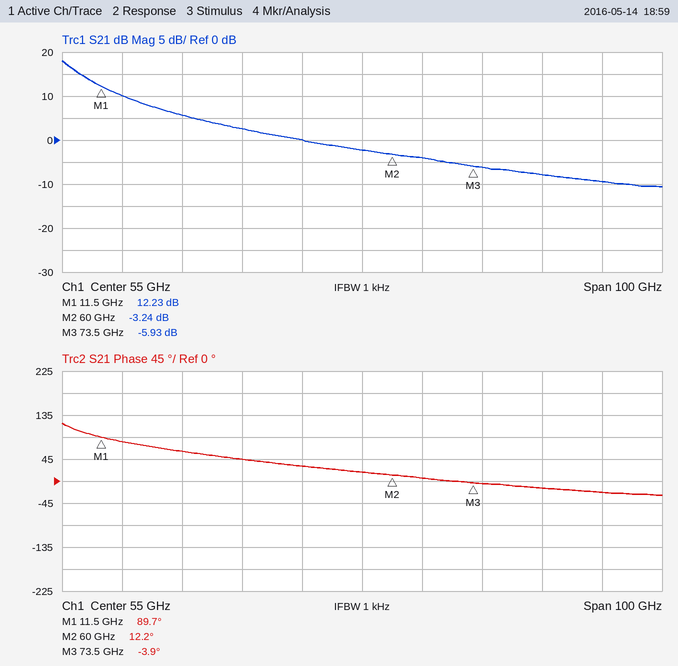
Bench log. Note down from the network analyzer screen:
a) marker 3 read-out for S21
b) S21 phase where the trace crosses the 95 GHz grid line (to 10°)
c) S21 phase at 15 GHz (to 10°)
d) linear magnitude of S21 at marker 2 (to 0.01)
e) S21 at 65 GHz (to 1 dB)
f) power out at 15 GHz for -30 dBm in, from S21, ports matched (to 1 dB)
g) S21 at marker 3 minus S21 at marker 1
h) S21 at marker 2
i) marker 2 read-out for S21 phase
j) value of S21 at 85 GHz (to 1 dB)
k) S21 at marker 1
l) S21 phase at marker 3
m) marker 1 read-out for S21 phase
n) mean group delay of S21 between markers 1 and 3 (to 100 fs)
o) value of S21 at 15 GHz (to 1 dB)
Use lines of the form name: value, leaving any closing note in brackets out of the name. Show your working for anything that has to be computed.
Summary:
marker 3 read-out for S21: -5.93 dB
S21 phase where the trace crosses the 95 GHz grid line: -20°
S21 phase at 15 GHz: 80°
linear magnitude of S21 at marker 2: 10^(-3.24/20) ≈ 0.69
S21 at 65 GHz: -4 dB
power out at 15 GHz for -30 dBm in, from S21, ports matched: -30 dBm + (10 dB) = -20 dBm
S21 at marker 3 minus S21 at marker 1: -5.93 − (12.23) = -18.16 dB
S21 at marker 2: -3.24 dB
marker 2 read-out for S21 phase: 12.2°
value of S21 at 85 GHz: -8 dB
S21 at marker 1: 12.23 dB
S21 phase at marker 3: -3.9°
marker 1 read-out for S21 phase: 89.7°
mean group delay of S21 between markers 1 and 3: −(-3.9° − (89.7°))/(360° × 62 GHz) ≈ 4.2 ps
value of S21 at 15 GHz: 10 dB
